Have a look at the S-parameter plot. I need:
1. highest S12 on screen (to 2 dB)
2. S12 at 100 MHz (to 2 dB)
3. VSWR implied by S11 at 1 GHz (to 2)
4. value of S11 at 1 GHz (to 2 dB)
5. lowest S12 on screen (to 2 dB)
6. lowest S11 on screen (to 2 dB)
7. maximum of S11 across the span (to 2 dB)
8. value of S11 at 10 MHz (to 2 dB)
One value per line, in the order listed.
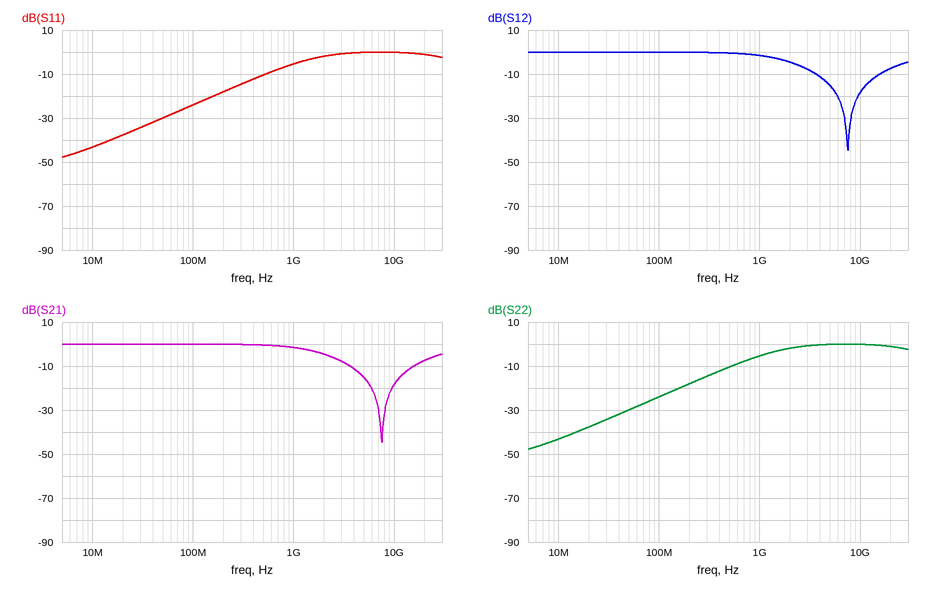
0 dB
0 dB
4
-6 dB
-44 dB
-48 dB
0 dB
-44 dB
